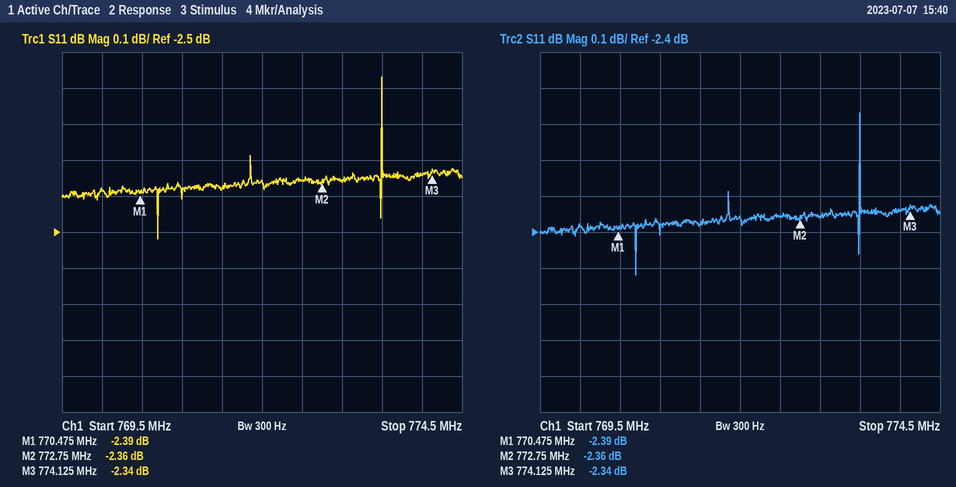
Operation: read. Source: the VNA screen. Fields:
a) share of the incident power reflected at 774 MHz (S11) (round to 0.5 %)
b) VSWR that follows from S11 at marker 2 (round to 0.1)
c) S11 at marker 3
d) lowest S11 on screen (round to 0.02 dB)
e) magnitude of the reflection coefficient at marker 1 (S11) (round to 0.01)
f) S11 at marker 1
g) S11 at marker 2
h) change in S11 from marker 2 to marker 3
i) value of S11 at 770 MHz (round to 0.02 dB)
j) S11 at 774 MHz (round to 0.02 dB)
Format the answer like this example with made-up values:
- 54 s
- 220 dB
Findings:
- 58.5 %
- 7.4
- -2.34 dB
- -2.52 dB
- 0.76
- -2.39 dB
- -2.36 dB
- 0.02 dB
- -2.38 dB
- -2.34 dB
